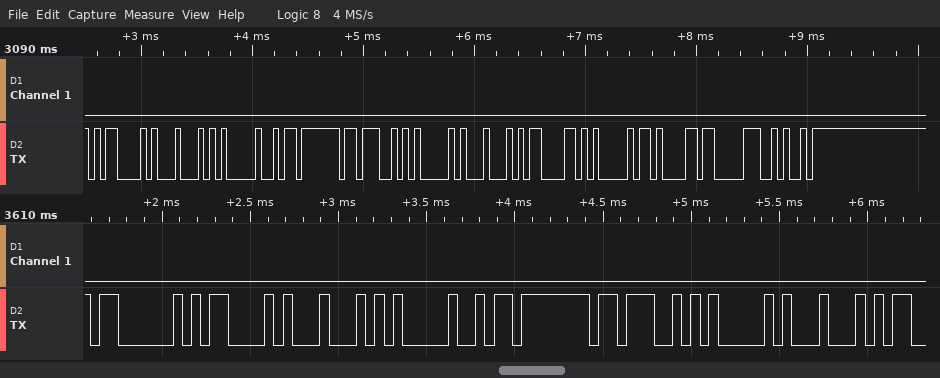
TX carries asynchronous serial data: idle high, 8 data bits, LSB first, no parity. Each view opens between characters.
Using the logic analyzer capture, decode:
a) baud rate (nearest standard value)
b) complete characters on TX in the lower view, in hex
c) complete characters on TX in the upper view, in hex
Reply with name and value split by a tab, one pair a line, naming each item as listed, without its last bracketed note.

baud rate	19200 baud
complete characters on TX in the lower view, in hex	03, 0D, 11, 05, DA, 3B, 05, 11
complete characters on TX in the upper view, in hex	0D, 11, 05, DA, 3B, 05, 11, 0D, 05, 0B, 83, 4A
